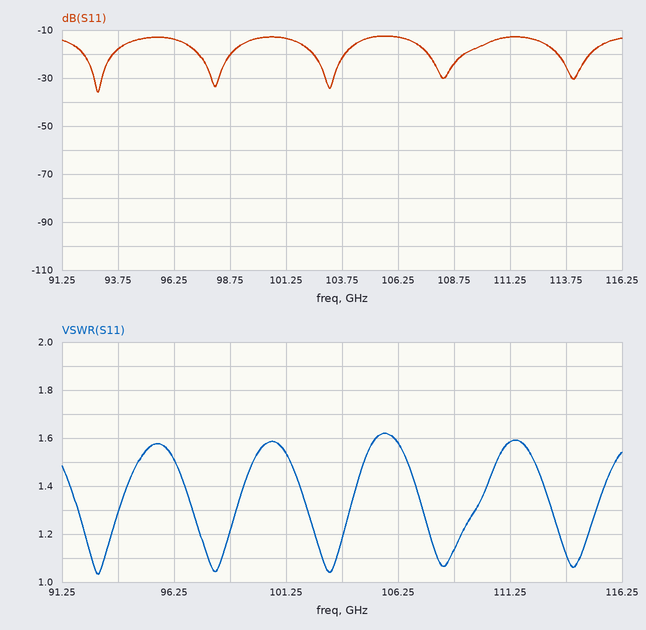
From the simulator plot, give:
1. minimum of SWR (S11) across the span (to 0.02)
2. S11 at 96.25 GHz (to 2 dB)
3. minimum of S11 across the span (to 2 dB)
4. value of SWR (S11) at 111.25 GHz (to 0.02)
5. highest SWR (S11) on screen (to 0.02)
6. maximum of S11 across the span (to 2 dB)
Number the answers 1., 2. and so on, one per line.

1. 1.04
2. -14 dB
3. -36 dB
4. 1.58
5. 1.62
6. -12 dB
